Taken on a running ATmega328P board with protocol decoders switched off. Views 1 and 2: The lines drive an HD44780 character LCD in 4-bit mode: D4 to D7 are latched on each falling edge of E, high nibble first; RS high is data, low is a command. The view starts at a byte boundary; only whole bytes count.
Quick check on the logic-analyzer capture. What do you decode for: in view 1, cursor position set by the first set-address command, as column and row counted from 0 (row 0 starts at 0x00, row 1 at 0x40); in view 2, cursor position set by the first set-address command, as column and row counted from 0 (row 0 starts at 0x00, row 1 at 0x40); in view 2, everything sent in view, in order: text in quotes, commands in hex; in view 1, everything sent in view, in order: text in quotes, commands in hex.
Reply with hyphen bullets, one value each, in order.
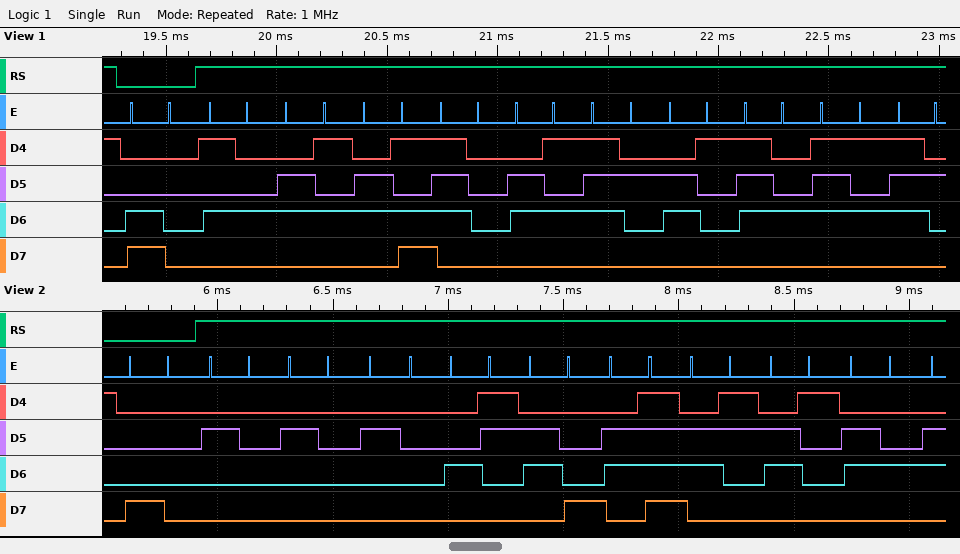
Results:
- column 0, row 1
- column 0, row 0
- 0x80 "   Chocad"
- 0xC0 "Temperatur"
